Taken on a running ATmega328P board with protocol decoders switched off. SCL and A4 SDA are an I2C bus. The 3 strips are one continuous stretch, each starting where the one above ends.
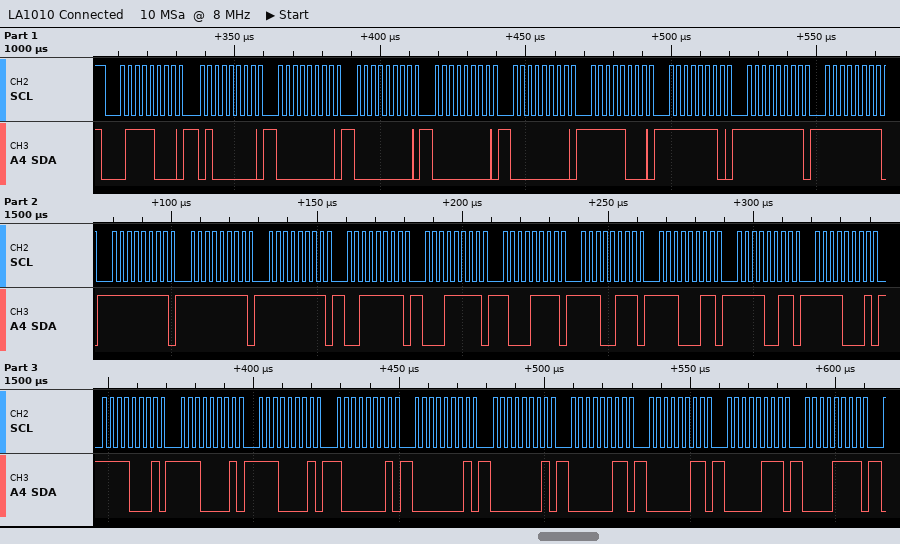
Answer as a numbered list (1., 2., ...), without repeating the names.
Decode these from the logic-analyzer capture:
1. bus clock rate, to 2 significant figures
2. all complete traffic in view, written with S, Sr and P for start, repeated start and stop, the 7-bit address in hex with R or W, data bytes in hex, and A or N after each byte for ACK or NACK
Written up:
1. 400 kHz
2. S 3CW A 40 A 00 A 00 A 00 A 00 A F8 A FE A FF A FF A FF A FF A FF A 3F A 1F A 8F A E7 A E3 A F3 A F1 A F1 A E1 A E1 A 81 A 01 A 01 A 03 A 03 A 07 A 0F A
